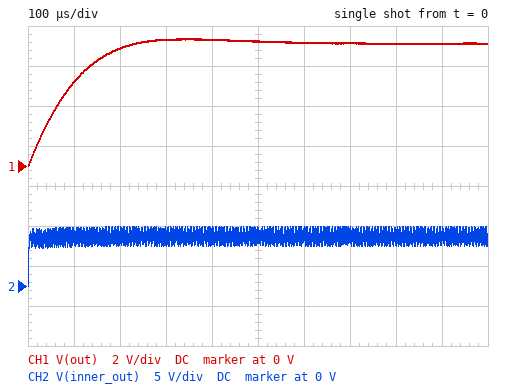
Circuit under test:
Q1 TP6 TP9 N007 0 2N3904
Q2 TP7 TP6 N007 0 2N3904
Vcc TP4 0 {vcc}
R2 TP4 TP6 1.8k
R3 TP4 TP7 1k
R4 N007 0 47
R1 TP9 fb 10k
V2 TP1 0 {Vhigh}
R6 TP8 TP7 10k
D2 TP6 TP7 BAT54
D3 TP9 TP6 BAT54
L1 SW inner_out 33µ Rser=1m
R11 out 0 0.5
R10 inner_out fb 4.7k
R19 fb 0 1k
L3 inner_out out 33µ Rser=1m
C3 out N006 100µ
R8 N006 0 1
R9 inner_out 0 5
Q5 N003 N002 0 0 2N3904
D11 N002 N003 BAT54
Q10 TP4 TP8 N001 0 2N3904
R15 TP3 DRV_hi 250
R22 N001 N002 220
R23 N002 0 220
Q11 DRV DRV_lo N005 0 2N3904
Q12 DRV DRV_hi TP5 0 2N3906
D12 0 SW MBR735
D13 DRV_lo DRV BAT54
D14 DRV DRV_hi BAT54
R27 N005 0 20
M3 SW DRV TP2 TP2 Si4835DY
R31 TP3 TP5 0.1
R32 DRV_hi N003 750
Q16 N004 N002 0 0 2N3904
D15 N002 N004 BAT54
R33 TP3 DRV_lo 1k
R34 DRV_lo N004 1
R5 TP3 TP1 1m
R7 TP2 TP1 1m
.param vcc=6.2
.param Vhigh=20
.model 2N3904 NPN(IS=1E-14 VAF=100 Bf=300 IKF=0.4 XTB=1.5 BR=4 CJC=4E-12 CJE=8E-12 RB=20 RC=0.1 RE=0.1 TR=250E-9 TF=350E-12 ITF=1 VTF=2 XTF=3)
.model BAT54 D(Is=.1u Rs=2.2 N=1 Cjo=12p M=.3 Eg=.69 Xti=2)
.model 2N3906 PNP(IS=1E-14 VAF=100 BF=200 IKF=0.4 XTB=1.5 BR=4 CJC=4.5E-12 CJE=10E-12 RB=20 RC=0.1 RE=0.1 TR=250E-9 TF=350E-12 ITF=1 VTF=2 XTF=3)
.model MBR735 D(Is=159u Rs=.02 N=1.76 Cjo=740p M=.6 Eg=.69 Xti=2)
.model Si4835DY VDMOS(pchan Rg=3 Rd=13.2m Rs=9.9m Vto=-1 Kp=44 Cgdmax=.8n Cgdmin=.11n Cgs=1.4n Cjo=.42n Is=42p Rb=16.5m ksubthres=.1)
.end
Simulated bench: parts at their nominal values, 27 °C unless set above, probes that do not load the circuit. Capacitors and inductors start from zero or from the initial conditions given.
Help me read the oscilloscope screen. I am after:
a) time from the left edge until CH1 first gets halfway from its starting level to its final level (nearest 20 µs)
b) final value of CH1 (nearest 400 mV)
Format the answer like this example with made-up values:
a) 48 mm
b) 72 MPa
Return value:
a) 60 µs
b) 6.0 V
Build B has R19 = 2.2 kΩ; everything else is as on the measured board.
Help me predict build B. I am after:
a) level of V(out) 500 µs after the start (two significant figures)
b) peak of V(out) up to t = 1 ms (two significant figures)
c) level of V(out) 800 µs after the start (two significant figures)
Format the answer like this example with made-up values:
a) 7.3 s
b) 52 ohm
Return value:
a) 3.6 V
b) 3.7 V
c) 3.5 V
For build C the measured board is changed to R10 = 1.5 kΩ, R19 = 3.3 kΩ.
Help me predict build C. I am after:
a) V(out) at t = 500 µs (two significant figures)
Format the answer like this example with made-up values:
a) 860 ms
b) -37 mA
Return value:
a) 1.8 V
